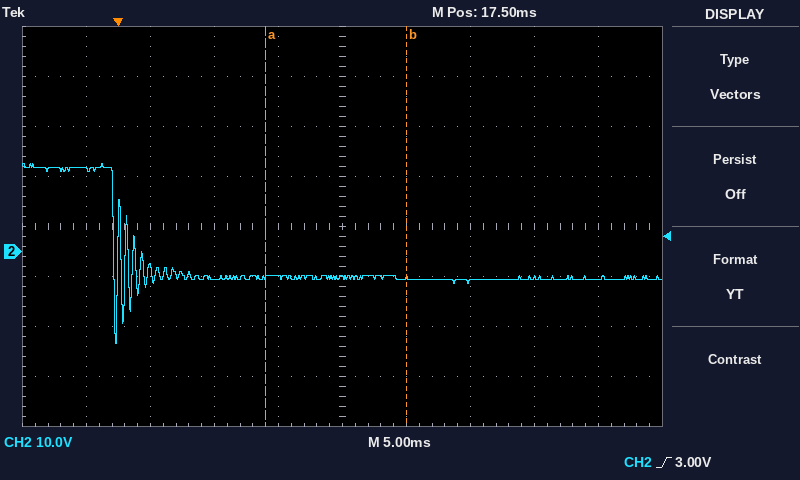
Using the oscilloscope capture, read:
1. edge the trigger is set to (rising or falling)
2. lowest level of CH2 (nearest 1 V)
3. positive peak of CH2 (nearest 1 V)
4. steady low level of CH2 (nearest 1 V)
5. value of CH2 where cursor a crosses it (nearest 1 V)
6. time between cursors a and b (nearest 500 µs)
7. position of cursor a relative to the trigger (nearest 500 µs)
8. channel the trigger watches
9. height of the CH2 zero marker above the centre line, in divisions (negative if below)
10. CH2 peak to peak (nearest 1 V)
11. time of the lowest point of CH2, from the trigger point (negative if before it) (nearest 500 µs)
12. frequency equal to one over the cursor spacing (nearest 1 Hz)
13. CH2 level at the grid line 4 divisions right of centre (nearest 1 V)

rising
-18 V
18 V
-6 V
-5 V
11.0 ms
+11.5 ms
CH2
-0.5 div
36 V
0.0 ms
91 Hz
-6 V
